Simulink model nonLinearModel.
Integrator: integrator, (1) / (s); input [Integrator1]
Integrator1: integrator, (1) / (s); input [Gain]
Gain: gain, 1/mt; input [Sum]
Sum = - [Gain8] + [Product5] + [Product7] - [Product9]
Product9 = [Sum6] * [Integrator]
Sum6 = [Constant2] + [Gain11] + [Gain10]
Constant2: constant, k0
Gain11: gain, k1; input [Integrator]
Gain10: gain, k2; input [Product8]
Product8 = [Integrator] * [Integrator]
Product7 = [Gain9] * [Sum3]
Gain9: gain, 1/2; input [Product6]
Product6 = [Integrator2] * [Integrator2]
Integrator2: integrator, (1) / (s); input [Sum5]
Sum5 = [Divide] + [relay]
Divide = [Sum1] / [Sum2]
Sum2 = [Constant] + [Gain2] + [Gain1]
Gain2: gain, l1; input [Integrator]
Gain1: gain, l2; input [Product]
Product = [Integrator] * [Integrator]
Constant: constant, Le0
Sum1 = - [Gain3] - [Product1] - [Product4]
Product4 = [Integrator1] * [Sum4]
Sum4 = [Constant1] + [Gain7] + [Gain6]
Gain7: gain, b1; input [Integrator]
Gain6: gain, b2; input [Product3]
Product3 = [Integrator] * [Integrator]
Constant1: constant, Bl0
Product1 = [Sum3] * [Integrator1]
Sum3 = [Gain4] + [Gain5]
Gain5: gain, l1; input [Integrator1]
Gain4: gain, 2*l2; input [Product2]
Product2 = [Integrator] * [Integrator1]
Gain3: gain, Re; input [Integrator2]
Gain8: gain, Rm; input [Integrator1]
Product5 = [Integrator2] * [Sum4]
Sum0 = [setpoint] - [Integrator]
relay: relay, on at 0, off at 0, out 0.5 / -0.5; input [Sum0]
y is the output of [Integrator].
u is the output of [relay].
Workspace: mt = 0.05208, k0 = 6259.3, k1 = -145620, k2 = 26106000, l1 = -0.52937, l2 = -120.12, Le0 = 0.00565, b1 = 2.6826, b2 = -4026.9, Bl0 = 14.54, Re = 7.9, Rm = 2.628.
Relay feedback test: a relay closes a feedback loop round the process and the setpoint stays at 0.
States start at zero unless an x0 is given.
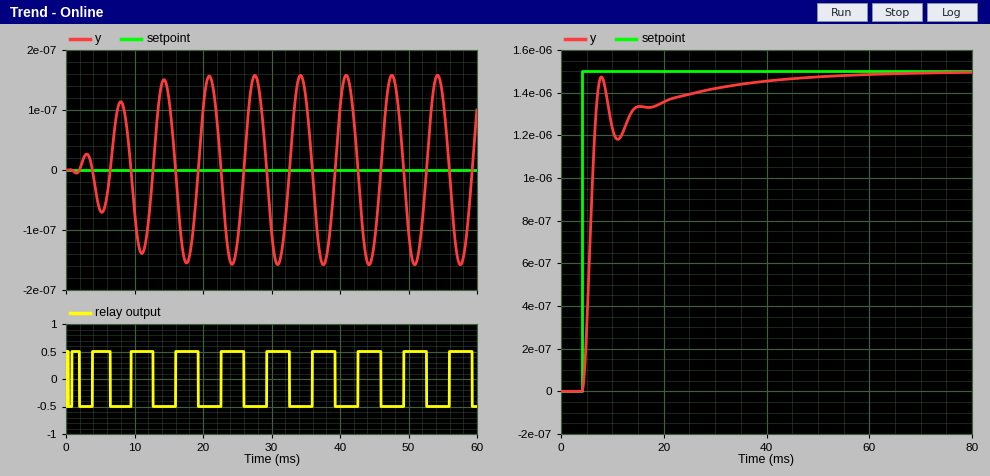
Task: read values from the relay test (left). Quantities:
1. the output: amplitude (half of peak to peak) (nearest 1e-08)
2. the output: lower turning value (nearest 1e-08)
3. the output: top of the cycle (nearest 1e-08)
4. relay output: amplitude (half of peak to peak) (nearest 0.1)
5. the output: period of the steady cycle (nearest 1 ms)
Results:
0.00000016
-0.00000016
0.00000016
0.5
7 ms
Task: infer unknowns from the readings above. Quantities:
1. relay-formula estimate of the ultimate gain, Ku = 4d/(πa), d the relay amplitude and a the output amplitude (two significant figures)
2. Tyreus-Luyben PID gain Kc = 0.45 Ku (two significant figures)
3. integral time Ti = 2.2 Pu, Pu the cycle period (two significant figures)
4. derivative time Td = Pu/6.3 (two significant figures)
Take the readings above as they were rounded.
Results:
4000000
1800000
15 ms
1.1 ms
